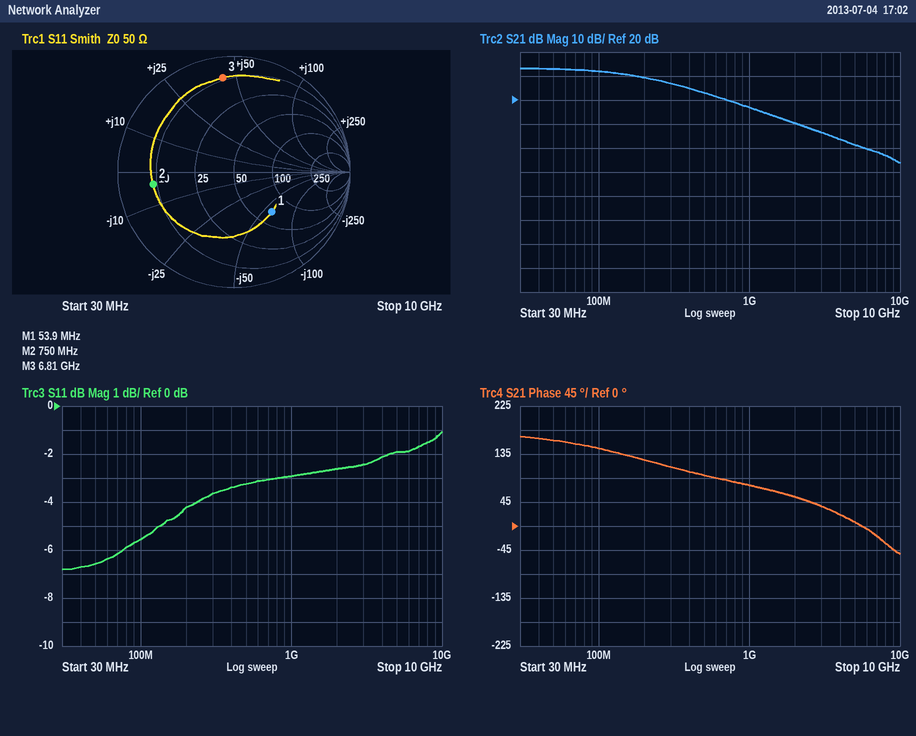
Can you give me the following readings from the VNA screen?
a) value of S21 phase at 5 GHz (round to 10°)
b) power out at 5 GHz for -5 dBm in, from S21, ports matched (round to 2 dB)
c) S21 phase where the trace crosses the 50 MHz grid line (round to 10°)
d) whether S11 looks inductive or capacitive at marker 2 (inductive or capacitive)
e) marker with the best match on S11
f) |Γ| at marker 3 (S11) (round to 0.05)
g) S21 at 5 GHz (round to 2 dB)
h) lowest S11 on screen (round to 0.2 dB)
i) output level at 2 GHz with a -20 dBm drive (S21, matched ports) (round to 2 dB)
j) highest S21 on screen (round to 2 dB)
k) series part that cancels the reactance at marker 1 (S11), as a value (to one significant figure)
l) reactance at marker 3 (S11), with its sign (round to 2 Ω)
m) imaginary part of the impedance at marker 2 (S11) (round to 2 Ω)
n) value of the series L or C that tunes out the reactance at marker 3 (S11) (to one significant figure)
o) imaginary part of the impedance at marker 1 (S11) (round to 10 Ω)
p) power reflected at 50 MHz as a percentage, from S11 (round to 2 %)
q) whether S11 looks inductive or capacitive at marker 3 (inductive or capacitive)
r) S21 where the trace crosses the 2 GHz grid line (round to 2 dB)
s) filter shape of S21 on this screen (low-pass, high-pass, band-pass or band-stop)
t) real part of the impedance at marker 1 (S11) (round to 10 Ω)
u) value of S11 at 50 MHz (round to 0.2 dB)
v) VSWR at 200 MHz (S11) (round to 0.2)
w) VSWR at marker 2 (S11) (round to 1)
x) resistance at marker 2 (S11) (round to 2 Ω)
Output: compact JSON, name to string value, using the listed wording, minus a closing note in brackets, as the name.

{"value of S21 phase at 5 GHz": "10°", "power out at 5 GHz for -5 dBm in, from S21, ports matched": "-4 dBm", "S21 phase where the trace crosses the 50 MHz grid line": "160°", "whether S11 looks inductive or capacitive at marker 2": "capacitive", "marker with the best match on S11": "marker 1", "|Γ| at marker 3 (S11)": "0.80", "S21 at 5 GHz": "2 dB", "lowest S11 on screen": "-6.8 dB", "output level at 2 GHz with a -20 dBm drive (S21, matched ports)": "-10 dBm", "highest S21 on screen": "34 dB", "series part that cancels the reactance at marker 1 (S11), as a value": "200 nH", "reactance at marker 3 (S11), with its sign": "+44 Ω", "imaginary part of the impedance at marker 2 (S11)": "-4 Ω", "value of the series L or C that tunes out the reactance at marker 3 (S11)": "500 fF", "imaginary part of the impedance at marker 1 (S11)": "-60 Ω", "power reflected at 50 MHz as a percentage, from S11": "22 %", "whether S11 looks inductive or capacitive at marker 3": "inductive", "S21 where the trace crosses the 2 GHz grid line": "10 dB", "filter shape of S21 on this screen": "low-pass", "real part of the impedance at marker 1 (S11)": "70 Ω", "value of S11 at 50 MHz": "-6.6 dB", "VSWR at 200 MHz (S11)": "4.2", "VSWR at marker 2 (S11)": "6", "resistance at marker 2 (S11)": "8 Ω"}
